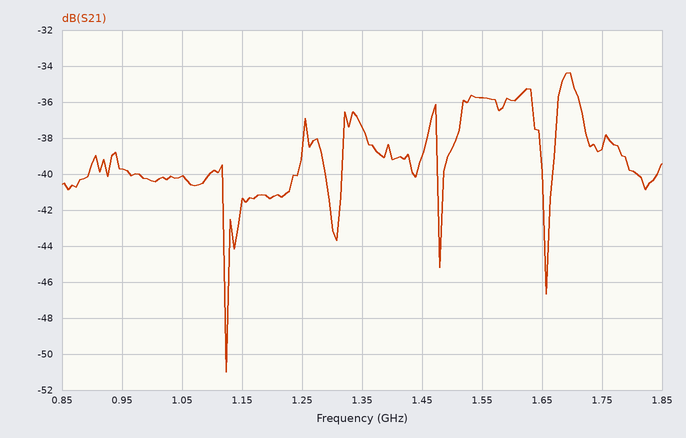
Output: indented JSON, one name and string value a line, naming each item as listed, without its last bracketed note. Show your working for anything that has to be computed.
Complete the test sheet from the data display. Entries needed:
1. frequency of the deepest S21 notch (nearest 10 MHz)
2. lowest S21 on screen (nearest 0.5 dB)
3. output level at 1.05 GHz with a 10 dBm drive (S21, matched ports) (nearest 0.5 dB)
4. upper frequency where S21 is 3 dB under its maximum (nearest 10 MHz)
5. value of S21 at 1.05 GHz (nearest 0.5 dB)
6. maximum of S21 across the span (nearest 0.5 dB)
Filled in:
{
  "frequency of the deepest S21 notch": "1.12 GHz",
  "lowest S21 on screen": "-51.0 dB",
  "output level at 1.05 GHz with a 10 dBm drive (S21, matched ports)": "10 dBm + (-40.0 dB) = -30.0 dBm",
  "upper frequency where S21 is 3 dB under its maximum": "1.72 GHz",
  "value of S21 at 1.05 GHz": "-40.0 dB",
  "maximum of S21 across the span": "-34.5 dB"
}
